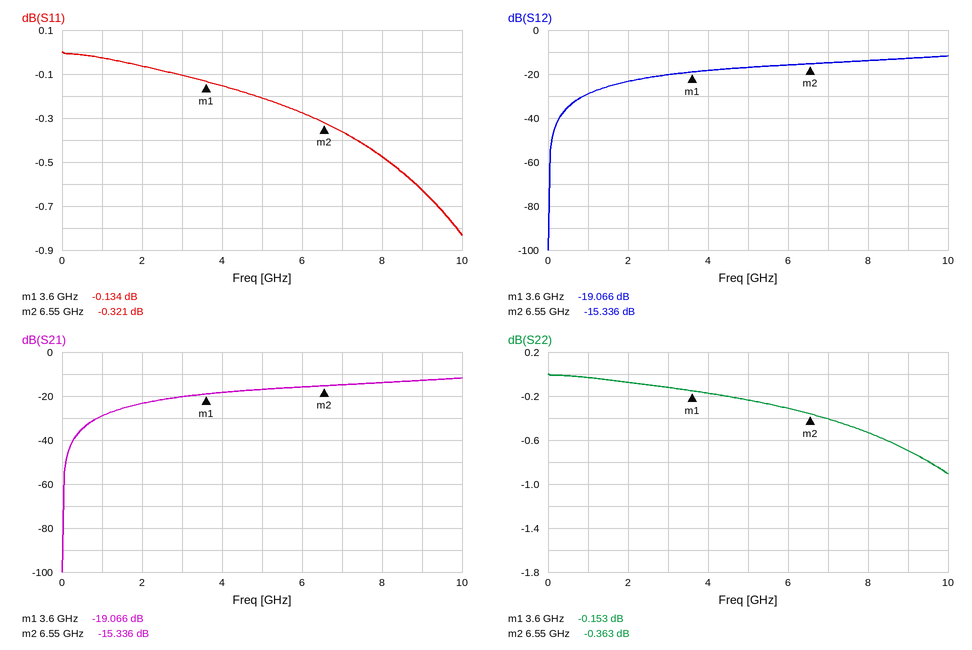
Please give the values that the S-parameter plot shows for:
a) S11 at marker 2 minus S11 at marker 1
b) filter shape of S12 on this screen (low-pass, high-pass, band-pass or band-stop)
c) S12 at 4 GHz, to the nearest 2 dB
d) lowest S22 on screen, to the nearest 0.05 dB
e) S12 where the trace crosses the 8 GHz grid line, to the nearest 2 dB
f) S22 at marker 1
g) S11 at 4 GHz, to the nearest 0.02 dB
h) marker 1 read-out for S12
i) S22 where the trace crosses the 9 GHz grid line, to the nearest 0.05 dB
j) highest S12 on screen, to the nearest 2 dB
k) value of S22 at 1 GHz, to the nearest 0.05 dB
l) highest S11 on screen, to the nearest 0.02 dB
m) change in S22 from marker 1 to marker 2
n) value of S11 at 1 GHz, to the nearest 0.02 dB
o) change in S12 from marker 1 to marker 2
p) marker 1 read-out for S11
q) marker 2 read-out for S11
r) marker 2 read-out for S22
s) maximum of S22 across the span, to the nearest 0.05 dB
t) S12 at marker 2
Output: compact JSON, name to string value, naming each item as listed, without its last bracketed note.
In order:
{"S11 at marker 2 minus S11 at marker 1": "-0.187 dB", "filter shape of S12 on this screen": "high-pass", "S12 at 4 GHz, to the nearest 2 dB": "-18 dB", "lowest S22 on screen, to the nearest 0.05 dB": "-0.90 dB", "S12 where the trace crosses the 8 GHz grid line, to the nearest 2 dB": "-14 dB", "S22 at marker 1": "-0.153 dB", "S11 at 4 GHz, to the nearest 0.02 dB": "-0.16 dB", "marker 1 read-out for S12": "-19.066 dB", "S22 where the trace crosses the 9 GHz grid line, to the nearest 0.05 dB": "-0.70 dB", "highest S12 on screen, to the nearest 2 dB": "-12 dB", "value of S22 at 1 GHz, to the nearest 0.05 dB": "-0.05 dB", "highest S11 on screen, to the nearest 0.02 dB": "0.00 dB", "change in S22 from marker 1 to marker 2": "-0.210 dB", "value of S11 at 1 GHz, to the nearest 0.02 dB": "-0.02 dB", "change in S12 from marker 1 to marker 2": "3.730 dB", "marker 1 read-out for S11": "-0.134 dB", "marker 2 read-out for S11": "-0.321 dB", "marker 2 read-out for S22": "-0.363 dB", "maximum of S22 across the span, to the nearest 0.05 dB": "0.00 dB", "S12 at marker 2": "-15.336 dB"}
